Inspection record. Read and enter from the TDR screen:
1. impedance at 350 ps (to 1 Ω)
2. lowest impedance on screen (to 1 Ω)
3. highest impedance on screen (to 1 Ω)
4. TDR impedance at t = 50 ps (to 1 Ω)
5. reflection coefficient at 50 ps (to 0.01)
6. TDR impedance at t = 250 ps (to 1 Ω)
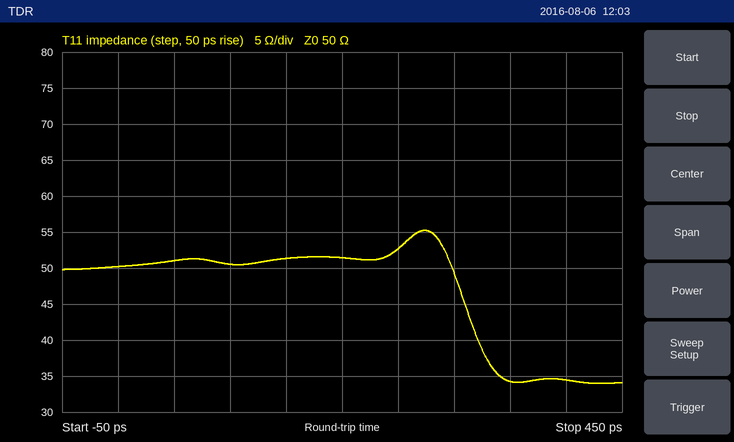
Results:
34 Ω
34 Ω
55 Ω
51 Ω
+0.01
53 Ω
